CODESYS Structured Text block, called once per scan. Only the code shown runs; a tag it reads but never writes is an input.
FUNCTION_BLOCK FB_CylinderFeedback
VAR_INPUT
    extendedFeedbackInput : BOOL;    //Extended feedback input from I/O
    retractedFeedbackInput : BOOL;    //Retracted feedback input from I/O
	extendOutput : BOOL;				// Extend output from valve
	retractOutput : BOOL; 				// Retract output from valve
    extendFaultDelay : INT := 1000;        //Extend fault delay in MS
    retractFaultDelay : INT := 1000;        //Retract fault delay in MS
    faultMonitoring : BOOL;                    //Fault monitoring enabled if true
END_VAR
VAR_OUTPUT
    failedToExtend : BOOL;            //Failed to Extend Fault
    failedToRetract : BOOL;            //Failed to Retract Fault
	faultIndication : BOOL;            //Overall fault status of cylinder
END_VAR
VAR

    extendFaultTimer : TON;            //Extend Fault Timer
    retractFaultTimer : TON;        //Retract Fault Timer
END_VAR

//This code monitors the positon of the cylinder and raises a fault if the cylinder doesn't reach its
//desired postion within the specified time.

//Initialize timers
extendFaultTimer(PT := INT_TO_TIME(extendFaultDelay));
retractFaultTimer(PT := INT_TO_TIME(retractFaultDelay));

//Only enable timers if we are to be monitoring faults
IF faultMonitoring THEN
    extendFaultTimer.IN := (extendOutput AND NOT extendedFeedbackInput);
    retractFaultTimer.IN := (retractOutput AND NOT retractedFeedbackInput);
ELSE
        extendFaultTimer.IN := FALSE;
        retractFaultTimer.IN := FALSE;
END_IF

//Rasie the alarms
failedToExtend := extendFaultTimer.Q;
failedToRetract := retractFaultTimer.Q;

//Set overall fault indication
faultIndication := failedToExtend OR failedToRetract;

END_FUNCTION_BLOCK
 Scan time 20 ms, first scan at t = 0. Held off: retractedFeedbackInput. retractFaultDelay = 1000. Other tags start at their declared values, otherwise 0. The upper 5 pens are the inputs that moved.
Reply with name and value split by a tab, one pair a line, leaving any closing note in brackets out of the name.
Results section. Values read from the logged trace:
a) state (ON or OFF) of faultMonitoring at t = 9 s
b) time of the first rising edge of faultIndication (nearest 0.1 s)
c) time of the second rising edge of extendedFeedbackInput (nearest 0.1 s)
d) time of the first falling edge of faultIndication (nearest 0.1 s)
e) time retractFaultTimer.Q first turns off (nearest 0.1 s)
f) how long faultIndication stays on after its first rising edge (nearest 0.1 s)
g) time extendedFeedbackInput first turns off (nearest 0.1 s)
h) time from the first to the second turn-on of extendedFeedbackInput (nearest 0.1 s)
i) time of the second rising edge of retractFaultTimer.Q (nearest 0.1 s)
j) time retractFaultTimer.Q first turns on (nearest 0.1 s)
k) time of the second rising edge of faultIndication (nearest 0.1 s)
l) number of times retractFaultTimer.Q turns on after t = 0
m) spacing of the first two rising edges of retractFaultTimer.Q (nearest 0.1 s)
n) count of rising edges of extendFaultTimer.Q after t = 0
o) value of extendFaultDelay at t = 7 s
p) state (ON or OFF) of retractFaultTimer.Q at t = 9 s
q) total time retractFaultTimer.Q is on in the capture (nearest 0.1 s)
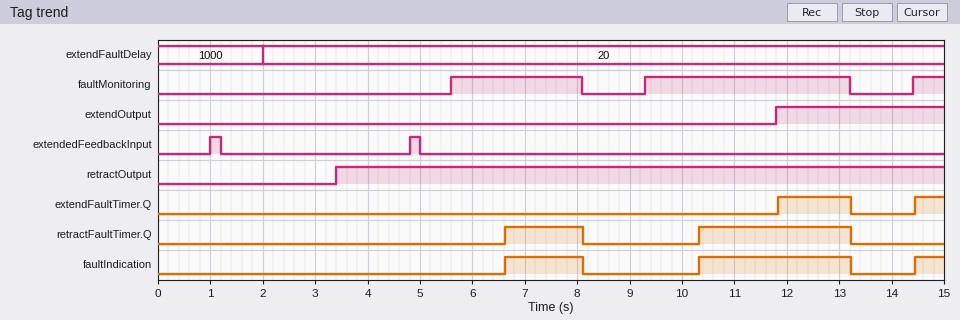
state (ON or OFF) of faultMonitoring at t = 9 s	OFF
time of the first rising edge of faultIndication	6.6 s
time of the second rising edge of extendedFeedbackInput	4.8 s
time of the first falling edge of faultIndication	8.1 s
time retractFaultTimer.Q first turns off	8.1 s
how long faultIndication stays on after its first rising edge	1.5 s
time extendedFeedbackInput first turns off	1.2 s
time from the first to the second turn-on of extendedFeedbackInput	3.8 s
time of the second rising edge of retractFaultTimer.Q	10.3 s
time retractFaultTimer.Q first turns on	6.6 s
time of the second rising edge of faultIndication	10.3 s
number of times retractFaultTimer.Q turns on after t = 0	2
spacing of the first two rising edges of retractFaultTimer.Q	3.7 s
count of rising edges of extendFaultTimer.Q after t = 0	2
value of extendFaultDelay at t = 7 s	20
state (ON or OFF) of retractFaultTimer.Q at t = 9 s	OFF
total time retractFaultTimer.Q is on in the capture	4.4 s
